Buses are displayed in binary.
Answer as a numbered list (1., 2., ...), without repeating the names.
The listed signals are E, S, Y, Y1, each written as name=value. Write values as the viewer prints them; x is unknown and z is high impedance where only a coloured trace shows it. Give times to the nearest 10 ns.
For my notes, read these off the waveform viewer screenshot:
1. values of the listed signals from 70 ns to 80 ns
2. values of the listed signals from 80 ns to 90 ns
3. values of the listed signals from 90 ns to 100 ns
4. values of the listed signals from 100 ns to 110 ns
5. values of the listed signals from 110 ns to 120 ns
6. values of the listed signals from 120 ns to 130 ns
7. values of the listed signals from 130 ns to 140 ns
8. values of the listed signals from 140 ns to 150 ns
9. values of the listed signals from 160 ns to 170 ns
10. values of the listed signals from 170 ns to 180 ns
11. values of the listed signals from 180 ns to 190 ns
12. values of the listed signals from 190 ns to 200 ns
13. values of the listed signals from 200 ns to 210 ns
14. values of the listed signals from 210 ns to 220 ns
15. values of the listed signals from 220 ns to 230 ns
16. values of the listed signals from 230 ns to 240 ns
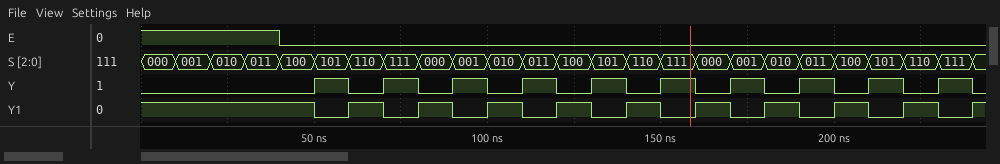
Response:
1. E=0, S=111, Y=1, Y1=0
2. E=0, S=000, Y=0, Y1=1
3. E=0, S=001, Y=1, Y1=0
4. E=0, S=010, Y=0, Y1=1
5. E=0, S=011, Y=1, Y1=0
6. E=0, S=100, Y=0, Y1=1
7. E=0, S=101, Y=1, Y1=0
8. E=0, S=110, Y=0, Y1=1
9. E=0, S=000, Y=0, Y1=1
10. E=0, S=001, Y=1, Y1=0
11. E=0, S=010, Y=0, Y1=1
12. E=0, S=011, Y=1, Y1=0
13. E=0, S=100, Y=0, Y1=1
14. E=0, S=101, Y=1, Y1=0
15. E=0, S=110, Y=0, Y1=1
16. E=0, S=111, Y=1, Y1=0
